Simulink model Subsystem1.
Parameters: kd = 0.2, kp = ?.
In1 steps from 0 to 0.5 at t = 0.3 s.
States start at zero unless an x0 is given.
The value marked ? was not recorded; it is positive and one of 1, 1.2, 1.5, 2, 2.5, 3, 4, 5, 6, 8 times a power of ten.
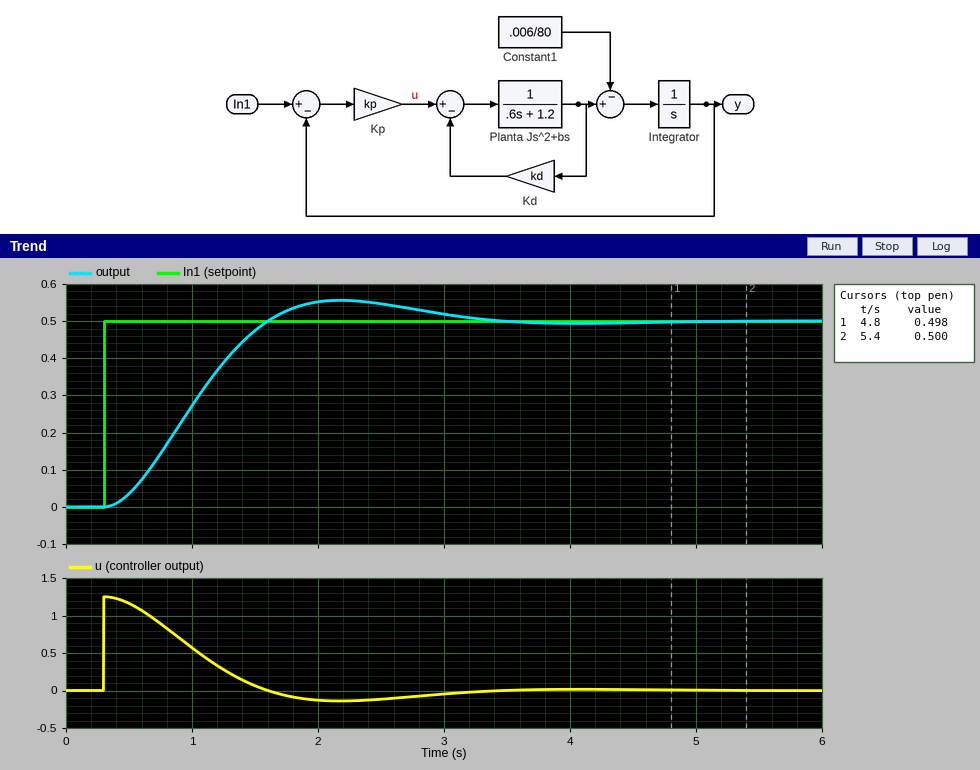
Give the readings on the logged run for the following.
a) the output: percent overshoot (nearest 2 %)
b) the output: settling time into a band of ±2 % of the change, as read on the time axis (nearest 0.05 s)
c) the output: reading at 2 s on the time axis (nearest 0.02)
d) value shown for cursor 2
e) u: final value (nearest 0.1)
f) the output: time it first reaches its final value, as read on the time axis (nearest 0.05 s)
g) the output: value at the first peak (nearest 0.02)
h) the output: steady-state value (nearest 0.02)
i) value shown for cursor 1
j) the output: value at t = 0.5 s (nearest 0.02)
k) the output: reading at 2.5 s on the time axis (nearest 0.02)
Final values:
12 %
3.20 s
0.56
0.500
0.0
1.60 s
0.56
0.50
0.498
0.04
0.54
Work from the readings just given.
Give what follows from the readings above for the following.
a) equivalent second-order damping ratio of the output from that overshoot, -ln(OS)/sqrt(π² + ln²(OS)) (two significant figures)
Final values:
0.56
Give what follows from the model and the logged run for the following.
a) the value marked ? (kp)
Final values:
2.5
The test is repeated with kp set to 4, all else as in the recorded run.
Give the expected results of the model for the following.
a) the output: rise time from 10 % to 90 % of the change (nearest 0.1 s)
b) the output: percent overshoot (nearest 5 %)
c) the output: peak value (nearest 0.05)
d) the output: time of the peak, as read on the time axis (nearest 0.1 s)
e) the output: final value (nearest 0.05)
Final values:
0.6 s
20 %
0.60
1.7 s
0.50
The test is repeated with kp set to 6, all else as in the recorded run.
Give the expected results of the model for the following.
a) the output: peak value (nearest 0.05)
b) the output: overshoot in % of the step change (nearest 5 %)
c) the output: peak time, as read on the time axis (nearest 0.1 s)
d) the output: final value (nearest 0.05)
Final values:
0.65
30 %
1.4 s
0.50
